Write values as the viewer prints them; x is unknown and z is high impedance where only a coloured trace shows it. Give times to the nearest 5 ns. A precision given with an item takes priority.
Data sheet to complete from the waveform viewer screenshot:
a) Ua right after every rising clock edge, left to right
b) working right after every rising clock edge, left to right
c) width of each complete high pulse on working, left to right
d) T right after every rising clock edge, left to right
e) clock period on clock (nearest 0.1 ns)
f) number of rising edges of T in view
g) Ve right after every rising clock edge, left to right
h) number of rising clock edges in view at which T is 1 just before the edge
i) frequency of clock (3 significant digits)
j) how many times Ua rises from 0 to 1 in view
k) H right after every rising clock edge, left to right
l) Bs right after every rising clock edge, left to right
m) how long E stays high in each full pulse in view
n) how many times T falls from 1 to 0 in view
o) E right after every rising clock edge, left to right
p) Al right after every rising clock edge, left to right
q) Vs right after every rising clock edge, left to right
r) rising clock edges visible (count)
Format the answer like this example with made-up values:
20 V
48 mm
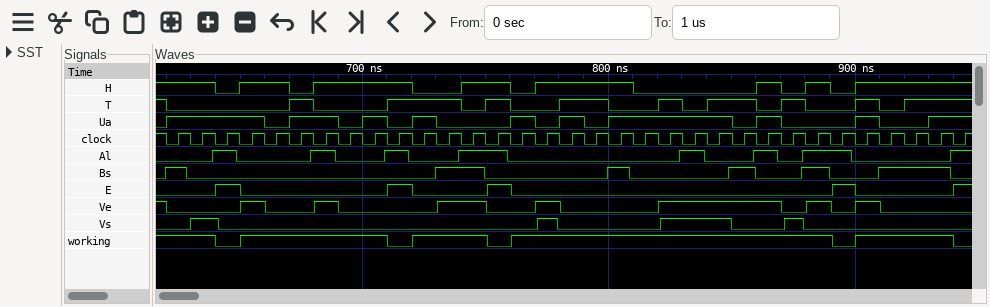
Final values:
1 1 1 1 0 1 1 0 1 0 1 0 0 0 1 0 1 0 1 1 1 1 1 0 1 0 0 0 1 0 0 1 1
1 1 0 1 1 1 1 1 1 0 1 1 1 0 1 1 1 1 1 1 1 1 1 1 1 1 1 0 1 1 1 1 0
60 ns, 30 ns, 130 ns, 40 ns
0 0 0 0 0 1 0 0 0 1 1 1 0 1 0 0 1 1 0 0 1 0 1 1 0 1 0 0 1 0 1 1 1
10 ns
9
0 0 0 1 0 0 1 0 0 0 0 1 1 0 0 1 0 0 0 0 1 1 1 1 1 0 1 0 1 0 0 0 0
15
100 MHz
10
1 1 0 1 1 0 1 1 1 1 0 0 1 1 0 1 1 1 1 0 0 0 0 0 1 0 1 0 1 1 1 1 1
1 0 0 0 0 0 0 0 0 0 0 1 1 0 0 0 0 0 1 0 0 0 0 1 0 0 1 0 0 1 1 1 0
10 ns, 10 ns, 10 ns, 10 ns
9
0 0 1 0 0 0 0 0 0 1 0 0 0 1 0 0 0 0 0 0 0 0 0 0 0 0 0 1 0 0 0 0 1
0 0 1 0 0 0 1 0 0 1 0 0 1 1 0 0 0 0 0 0 0 1 0 0 1 0 1 1 0 0 0 0 1
0 1 0 0 0 0 0 0 0 0 0 0 0 0 0 1 0 0 0 0 1 1 1 0 0 1 0 0 0 0 0 0 0
33
